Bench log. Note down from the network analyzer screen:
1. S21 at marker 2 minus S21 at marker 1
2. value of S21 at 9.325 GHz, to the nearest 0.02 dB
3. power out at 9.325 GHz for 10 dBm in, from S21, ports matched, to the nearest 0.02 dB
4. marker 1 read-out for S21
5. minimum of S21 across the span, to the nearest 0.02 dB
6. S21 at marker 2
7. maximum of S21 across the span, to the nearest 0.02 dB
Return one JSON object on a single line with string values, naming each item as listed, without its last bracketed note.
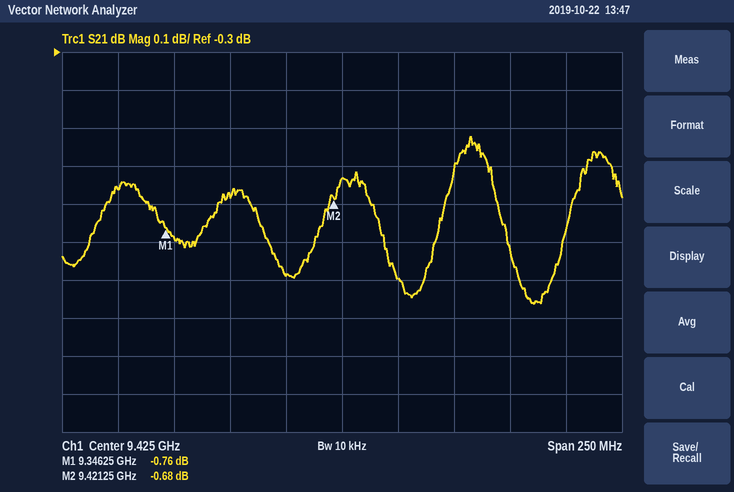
{"S21 at marker 2 minus S21 at marker 1": "0.08 dB", "value of S21 at 9.325 GHz, to the nearest 0.02 dB": "-0.66 dB", "power out at 9.325 GHz for 10 dBm in, from S21, ports matched, to the nearest 0.02 dB": "9.34 dBm", "marker 1 read-out for S21": "-0.76 dB", "minimum of S21 across the span, to the nearest 0.02 dB": "-0.96 dB", "S21 at marker 2": "-0.68 dB", "maximum of S21 across the span, to the nearest 0.02 dB": "-0.52 dB"}
